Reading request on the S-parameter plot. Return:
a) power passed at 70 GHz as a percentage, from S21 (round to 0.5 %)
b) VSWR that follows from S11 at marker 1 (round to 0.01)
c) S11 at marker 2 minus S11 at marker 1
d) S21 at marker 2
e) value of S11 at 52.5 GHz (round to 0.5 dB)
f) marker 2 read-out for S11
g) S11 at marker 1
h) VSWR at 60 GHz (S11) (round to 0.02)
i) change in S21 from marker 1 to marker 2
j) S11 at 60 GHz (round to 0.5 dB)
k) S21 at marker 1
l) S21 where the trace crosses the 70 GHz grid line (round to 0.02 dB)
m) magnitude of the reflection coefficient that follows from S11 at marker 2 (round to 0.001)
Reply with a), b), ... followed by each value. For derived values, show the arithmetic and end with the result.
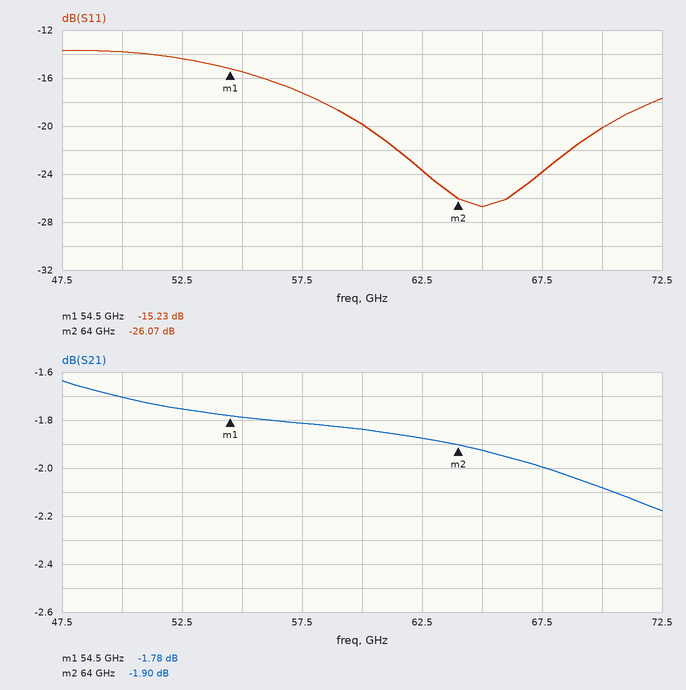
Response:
a) 10^(-2.08/10) ≈ 61.9 %, so 62.0 % to the nearest 0.5 %
b) (1 + 0.1732)/(1 − 0.1732) ≈ 1.42
c) -26.07 − (-15.23) = -10.84 dB
d) -1.90 dB
e) -14.5 dB
f) -26.07 dB
g) -15.23 dB
h) |Γ| = 10^(-20/20) = 0.1000; VSWR = (1 + 0.1000)/(1 − 0.1000) ≈ 1.22
i) -1.9 − (-1.78) = -0.12 dB
j) -20.0 dB
k) -1.78 dB
l) -2.08 dB
m) 10^(-26.07/20) ≈ 0.050
